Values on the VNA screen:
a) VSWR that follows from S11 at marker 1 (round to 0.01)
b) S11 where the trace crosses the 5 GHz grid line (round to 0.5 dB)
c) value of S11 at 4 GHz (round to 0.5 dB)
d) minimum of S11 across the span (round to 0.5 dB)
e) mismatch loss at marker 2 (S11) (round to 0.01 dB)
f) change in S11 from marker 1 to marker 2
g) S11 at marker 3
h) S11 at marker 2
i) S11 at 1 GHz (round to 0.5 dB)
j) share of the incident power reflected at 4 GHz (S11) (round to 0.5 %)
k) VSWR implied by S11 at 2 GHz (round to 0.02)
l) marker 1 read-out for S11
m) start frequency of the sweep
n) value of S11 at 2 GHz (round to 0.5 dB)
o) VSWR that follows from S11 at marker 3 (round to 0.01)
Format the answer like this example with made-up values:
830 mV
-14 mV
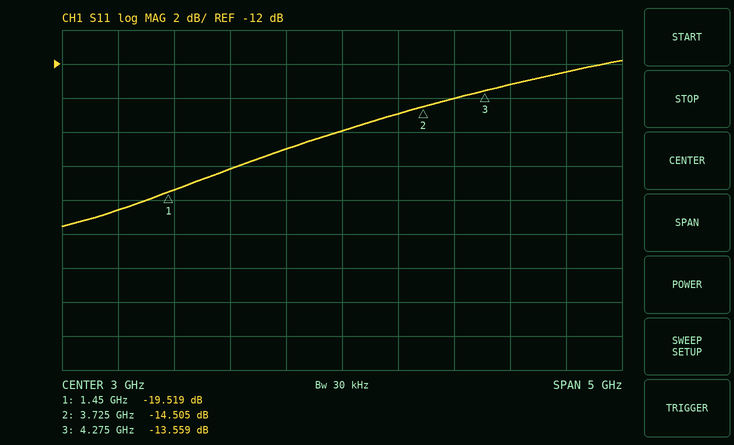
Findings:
1.24
-12.5 dB
-14.0 dB
-21.5 dB
0.16 dB
5.014 dB
-13.559 dB
-14.505 dB
-20.5 dB
4.0 %
1.28
-19.519 dB
500 MHz
-18.0 dB
1.53
